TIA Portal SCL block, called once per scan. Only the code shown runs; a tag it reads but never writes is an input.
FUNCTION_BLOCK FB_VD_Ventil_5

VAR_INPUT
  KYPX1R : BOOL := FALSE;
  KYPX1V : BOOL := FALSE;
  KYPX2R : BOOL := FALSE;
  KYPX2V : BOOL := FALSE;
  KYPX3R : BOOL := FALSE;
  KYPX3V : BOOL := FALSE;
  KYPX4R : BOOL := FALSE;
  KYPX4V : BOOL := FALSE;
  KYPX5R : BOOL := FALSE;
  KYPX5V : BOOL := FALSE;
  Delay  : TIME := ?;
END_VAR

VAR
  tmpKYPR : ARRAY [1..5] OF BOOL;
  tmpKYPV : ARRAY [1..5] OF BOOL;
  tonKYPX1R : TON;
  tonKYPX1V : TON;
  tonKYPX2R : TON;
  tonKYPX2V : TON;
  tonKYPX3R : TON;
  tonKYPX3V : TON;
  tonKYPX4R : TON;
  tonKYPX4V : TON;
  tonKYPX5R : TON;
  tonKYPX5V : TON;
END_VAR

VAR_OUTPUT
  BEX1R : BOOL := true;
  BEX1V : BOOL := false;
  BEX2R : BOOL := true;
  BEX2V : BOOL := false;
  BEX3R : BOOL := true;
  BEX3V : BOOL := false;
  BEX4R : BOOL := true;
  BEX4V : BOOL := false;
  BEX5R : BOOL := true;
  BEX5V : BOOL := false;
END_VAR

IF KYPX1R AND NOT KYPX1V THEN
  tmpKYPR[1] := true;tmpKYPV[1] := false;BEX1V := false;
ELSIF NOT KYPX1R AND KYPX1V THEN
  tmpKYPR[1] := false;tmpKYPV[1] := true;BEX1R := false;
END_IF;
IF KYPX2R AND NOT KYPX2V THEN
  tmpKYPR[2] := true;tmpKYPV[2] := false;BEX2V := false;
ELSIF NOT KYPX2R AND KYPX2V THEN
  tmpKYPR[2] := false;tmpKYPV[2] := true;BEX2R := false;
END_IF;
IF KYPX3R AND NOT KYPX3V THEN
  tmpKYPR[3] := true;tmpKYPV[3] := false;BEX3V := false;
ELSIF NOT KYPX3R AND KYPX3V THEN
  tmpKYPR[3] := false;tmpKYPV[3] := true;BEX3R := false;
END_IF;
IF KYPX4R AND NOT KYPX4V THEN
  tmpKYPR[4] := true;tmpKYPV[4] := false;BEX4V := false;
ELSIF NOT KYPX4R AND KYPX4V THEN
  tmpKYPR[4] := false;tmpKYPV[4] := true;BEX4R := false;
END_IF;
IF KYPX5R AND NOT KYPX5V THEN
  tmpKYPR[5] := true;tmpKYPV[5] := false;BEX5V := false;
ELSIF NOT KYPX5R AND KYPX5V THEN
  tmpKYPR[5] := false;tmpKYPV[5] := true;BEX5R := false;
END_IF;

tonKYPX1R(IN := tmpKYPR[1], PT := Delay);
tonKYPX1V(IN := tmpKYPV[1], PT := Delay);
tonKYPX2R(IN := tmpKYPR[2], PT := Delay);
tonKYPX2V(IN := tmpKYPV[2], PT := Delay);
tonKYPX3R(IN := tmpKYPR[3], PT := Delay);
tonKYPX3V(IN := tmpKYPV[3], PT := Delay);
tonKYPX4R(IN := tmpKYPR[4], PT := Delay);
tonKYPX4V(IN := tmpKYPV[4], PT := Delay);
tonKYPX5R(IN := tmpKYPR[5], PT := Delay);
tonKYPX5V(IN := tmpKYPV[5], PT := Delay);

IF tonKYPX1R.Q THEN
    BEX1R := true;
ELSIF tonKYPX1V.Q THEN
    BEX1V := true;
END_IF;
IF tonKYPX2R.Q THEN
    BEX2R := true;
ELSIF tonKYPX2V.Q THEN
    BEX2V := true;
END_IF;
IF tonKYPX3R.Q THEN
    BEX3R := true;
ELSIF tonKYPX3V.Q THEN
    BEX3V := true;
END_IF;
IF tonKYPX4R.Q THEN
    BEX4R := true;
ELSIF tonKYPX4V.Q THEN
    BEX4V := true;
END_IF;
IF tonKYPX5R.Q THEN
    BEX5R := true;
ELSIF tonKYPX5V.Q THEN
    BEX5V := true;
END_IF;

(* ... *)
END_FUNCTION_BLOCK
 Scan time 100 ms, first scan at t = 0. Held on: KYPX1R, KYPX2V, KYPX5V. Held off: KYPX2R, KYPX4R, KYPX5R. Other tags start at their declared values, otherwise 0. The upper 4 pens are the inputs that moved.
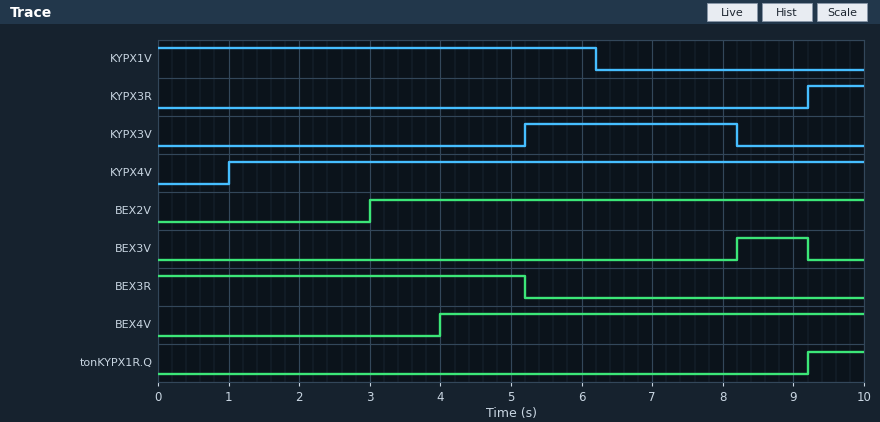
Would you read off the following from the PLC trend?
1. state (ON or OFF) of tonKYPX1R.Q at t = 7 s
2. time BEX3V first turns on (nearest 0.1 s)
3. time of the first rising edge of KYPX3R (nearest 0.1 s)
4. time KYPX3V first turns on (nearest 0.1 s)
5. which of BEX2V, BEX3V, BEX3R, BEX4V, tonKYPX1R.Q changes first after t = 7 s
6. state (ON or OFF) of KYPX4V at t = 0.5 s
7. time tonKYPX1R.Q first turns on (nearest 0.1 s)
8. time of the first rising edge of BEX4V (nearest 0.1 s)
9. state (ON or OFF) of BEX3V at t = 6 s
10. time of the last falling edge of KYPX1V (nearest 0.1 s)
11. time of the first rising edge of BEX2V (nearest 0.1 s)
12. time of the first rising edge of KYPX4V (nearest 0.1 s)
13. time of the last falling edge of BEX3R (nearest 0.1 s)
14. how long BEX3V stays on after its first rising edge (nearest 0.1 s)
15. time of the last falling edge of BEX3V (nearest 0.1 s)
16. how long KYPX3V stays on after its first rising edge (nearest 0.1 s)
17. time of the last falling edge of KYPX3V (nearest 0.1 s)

OFF
8.2 s
9.2 s
5.2 s
BEX3V
OFF
9.2 s
4.0 s
OFF
6.2 s
3.0 s
1.0 s
5.2 s
1.0 s
9.2 s
3.0 s
8.2 s
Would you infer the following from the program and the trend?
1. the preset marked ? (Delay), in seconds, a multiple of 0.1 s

3.0 s
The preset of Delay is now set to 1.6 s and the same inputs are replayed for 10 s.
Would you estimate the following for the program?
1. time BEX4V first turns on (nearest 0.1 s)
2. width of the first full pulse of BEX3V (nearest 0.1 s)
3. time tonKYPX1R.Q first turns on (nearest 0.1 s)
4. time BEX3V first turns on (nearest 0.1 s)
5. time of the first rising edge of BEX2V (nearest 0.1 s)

2.6 s
2.4 s
7.8 s
6.8 s
1.6 s
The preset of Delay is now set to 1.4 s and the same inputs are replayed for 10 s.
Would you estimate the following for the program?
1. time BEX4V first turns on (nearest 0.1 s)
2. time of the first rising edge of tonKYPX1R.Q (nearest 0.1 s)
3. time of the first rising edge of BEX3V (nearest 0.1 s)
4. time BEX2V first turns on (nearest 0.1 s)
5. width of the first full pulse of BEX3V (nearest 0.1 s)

2.4 s
7.6 s
6.6 s
1.4 s
2.6 s
